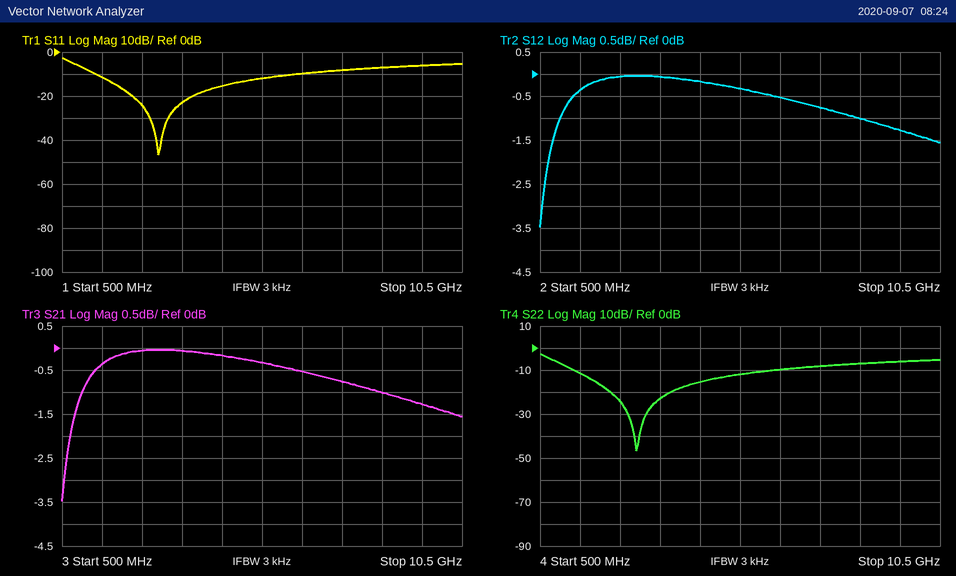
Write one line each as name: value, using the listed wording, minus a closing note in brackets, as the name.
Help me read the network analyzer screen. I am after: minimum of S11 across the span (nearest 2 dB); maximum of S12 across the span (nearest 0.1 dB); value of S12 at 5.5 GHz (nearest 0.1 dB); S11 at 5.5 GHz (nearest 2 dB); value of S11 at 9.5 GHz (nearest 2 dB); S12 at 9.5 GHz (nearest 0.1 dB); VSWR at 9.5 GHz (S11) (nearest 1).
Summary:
minimum of S11 across the span: -46 dB
maximum of S12 across the span: 0.0 dB
value of S12 at 5.5 GHz: -0.3 dB
S11 at 5.5 GHz: -12 dB
value of S11 at 9.5 GHz: -6 dB
S12 at 9.5 GHz: -1.3 dB
VSWR at 9.5 GHz (S11): 3
